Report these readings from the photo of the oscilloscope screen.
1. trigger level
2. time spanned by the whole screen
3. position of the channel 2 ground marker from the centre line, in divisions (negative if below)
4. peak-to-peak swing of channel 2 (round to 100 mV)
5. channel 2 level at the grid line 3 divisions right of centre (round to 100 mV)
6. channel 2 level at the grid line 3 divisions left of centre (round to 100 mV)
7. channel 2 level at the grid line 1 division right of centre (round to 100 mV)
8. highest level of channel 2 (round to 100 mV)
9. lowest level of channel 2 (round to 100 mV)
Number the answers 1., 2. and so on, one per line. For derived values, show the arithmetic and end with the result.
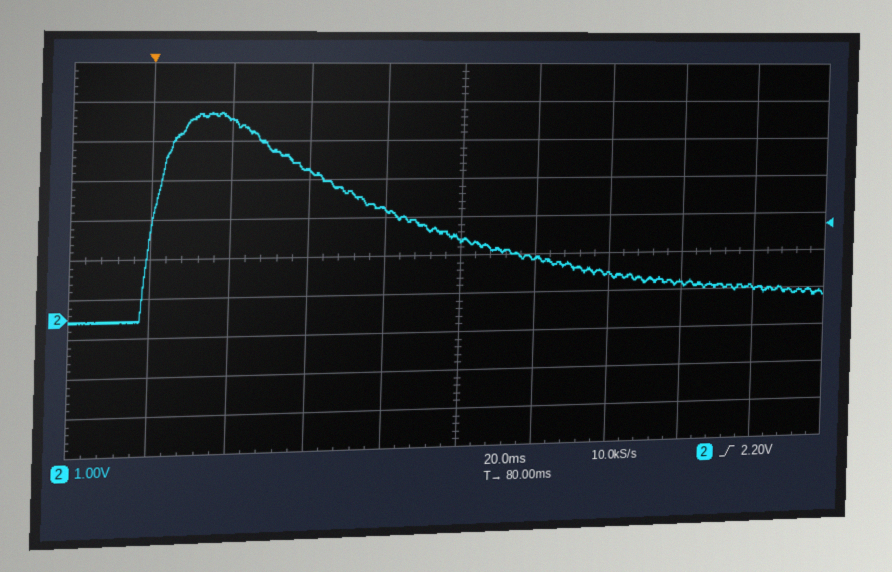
1. 2.20 V
2. 200 ms
3. -1.5 div
4. 5.2 V − (-100 mV) = 5.3 V
5. 700 mV
6. 5.1 V
7. 1.4 V
8. 5.2 V
9. -100 mV
